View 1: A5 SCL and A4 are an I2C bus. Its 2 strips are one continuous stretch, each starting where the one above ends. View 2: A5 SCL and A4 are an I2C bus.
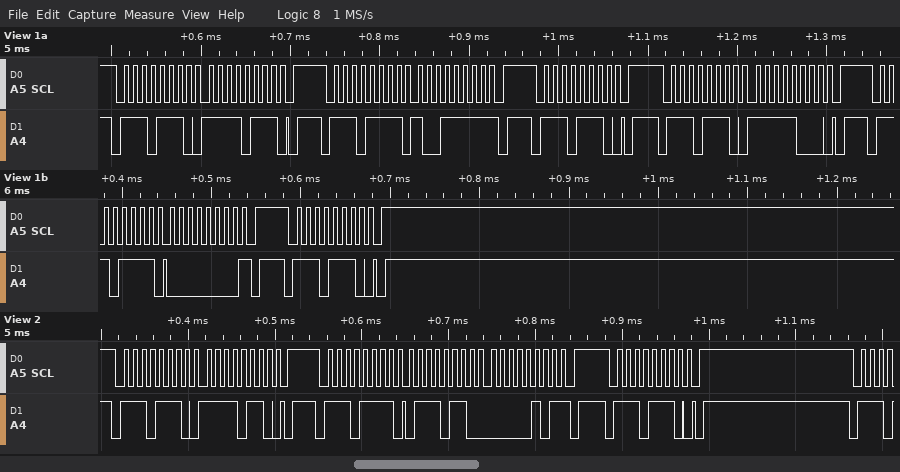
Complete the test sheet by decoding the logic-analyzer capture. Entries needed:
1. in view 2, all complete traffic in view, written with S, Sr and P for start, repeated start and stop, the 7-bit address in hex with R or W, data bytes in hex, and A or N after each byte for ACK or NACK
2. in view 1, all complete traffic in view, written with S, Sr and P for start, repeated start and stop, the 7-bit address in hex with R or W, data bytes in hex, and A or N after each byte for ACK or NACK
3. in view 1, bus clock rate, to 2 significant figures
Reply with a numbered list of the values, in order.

1. S 77W A F6 A P S 77R A 76 A 05 N P S 77W A P
2. S 77W A F7 A P S 77R A 9F N P S 77W A P S 77W A F8 A P S 77R A 00 N P S 77W A P
3. 100 kHz
